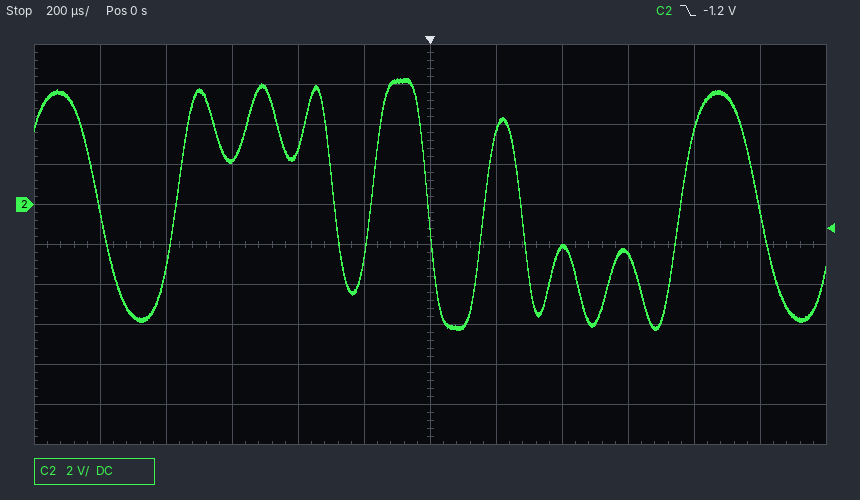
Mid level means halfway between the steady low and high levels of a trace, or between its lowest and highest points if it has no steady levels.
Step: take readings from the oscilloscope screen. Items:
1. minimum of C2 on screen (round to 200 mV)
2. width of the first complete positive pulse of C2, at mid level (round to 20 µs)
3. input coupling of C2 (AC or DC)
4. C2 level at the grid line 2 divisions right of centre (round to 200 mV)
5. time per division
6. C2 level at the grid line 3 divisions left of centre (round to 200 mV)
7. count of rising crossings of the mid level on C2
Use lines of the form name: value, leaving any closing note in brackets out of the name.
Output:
minimum of C2 on screen: -6.2 V
width of the first complete positive pulse of C2, at mid level: 480 µs
input coupling of C2: DC
C2 level at the grid line 2 divisions right of centre: -2.2 V
time per division: 200 µs
C2 level at the grid line 3 divisions left of centre: 2.2 V
count of rising crossings of the mid level on C2: 4
